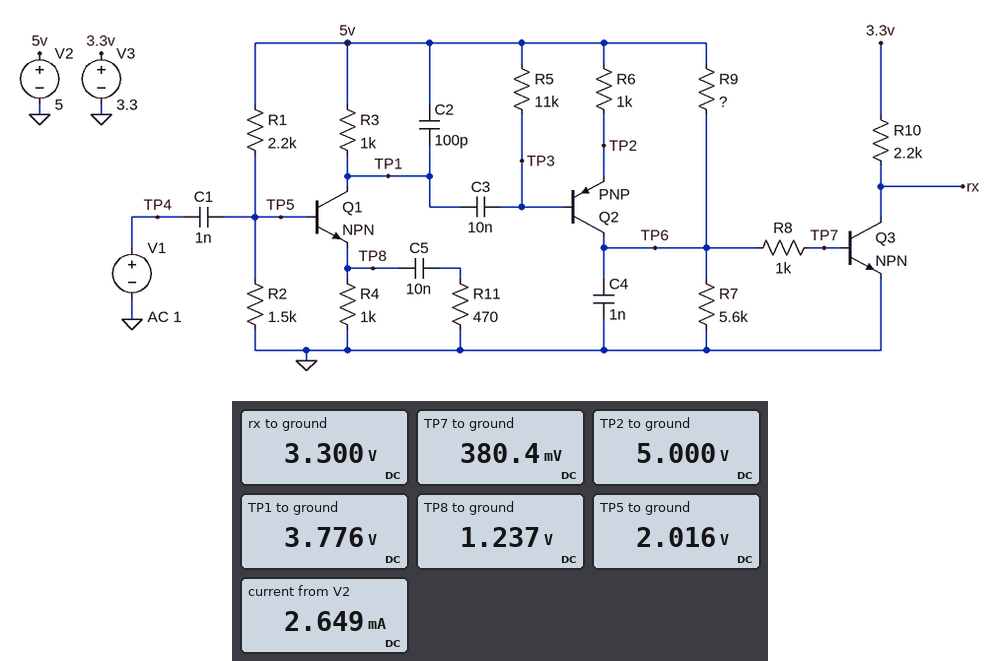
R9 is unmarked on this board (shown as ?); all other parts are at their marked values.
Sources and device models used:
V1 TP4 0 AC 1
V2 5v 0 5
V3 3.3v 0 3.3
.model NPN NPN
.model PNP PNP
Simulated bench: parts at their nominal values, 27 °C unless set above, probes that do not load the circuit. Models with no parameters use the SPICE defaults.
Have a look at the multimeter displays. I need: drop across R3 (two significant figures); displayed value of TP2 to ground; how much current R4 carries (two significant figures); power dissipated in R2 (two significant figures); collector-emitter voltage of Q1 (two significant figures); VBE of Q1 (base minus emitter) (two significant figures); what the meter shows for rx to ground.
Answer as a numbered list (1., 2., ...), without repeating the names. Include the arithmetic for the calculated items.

1. 5 V - 3.776 V = 1.2 V
2. 5.000 V
3. (1.237 V) / 1 kΩ = 1.2 mA
4. (2.016 V)^2 / 1.5 kΩ = 2.7 mW
5. 3.776 V - 1.237 V = 2.5 V
6. 2.016 V - 1.237 V = 780 mV
7. 3.300 V
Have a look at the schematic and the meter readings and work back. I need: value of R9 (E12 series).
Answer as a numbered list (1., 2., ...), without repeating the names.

1. 68 kΩ
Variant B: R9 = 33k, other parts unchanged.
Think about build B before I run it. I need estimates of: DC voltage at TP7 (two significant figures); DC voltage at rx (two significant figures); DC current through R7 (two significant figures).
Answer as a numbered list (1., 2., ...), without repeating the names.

1. 720 mV
2. 3.0 V
3. 130 µA
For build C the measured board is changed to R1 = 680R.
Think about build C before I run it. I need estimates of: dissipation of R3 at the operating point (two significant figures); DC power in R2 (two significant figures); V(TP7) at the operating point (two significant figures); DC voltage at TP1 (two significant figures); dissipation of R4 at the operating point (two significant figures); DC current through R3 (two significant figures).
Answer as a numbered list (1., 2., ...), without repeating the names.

1. 5.6 mW
2. 7.5 mW
3. 380 mV
4. 2.6 V
5. 6.5 mW
6. 2.4 mA
